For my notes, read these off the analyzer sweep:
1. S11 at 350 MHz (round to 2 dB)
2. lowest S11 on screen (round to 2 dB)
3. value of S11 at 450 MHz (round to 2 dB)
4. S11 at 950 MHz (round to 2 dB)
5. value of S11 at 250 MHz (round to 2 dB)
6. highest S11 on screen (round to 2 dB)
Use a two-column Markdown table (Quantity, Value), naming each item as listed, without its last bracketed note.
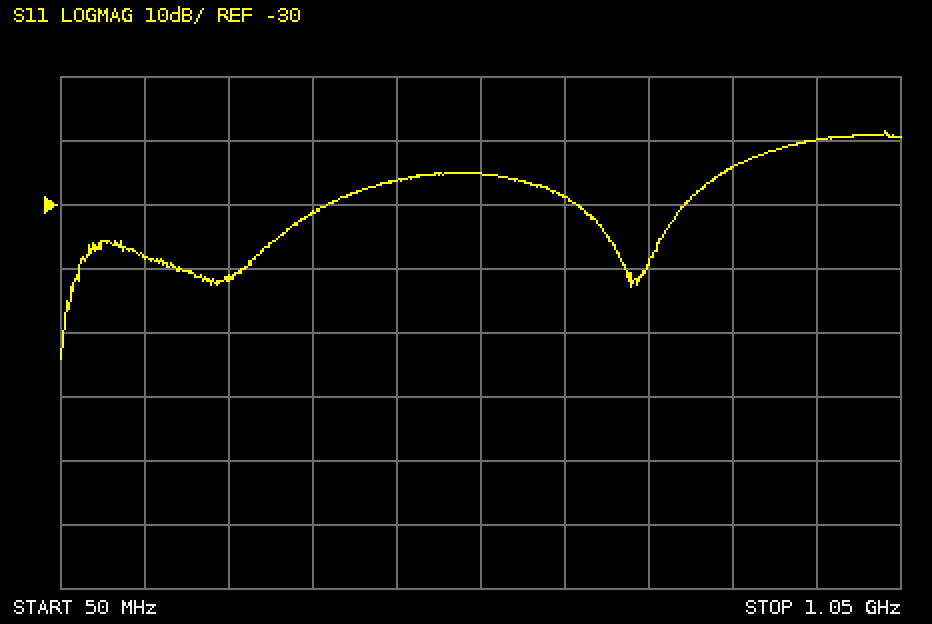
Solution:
| Quantity | Value |
|---|---|
| S11 at 350 MHz | -32 dB |
| lowest S11 on screen | -54 dB |
| value of S11 at 450 MHz | -26 dB |
| S11 at 950 MHz | -20 dB |
| value of S11 at 250 MHz | -42 dB |
| highest S11 on screen | -18 dB |
